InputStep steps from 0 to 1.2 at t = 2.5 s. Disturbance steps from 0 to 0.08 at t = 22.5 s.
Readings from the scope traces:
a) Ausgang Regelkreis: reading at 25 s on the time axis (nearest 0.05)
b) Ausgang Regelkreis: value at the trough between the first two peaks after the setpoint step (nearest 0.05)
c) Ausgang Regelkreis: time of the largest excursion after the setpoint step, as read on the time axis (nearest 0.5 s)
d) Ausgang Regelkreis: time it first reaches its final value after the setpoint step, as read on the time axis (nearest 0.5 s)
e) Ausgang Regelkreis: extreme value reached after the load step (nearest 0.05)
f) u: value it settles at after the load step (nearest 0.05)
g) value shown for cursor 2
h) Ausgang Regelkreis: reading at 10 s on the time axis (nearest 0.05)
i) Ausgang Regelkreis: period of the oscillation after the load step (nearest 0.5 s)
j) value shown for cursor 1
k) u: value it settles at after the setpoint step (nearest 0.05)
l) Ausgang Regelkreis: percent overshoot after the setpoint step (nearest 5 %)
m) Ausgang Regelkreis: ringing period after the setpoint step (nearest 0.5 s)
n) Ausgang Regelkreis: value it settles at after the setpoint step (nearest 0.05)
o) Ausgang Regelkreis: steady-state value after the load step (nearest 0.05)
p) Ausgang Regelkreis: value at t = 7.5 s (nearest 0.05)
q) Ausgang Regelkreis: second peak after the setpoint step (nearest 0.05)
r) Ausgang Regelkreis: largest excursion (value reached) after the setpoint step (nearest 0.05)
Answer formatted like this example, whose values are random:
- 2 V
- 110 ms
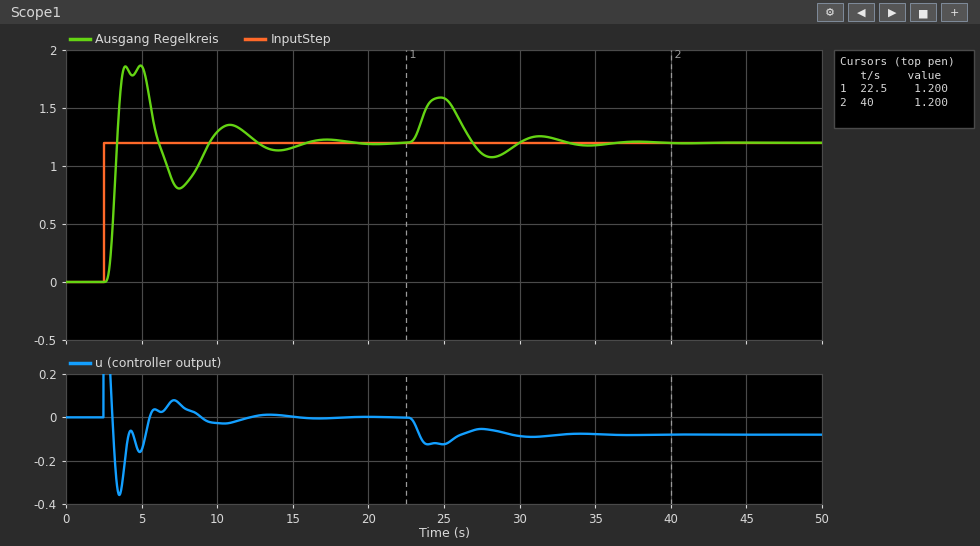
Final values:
- 1.60
- 0.80
- 5.0 s
- 3.5 s
- 1.60
- -0.10
- 1.200
- 1.30
- 6.5 s
- 1.200
- 0.00
- 55 %
- 6.0 s
- 1.20
- 1.20
- 0.80
- 1.35
- 1.85
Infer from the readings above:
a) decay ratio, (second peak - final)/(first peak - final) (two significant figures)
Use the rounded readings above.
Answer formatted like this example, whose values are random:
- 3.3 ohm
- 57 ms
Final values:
- 0.23
